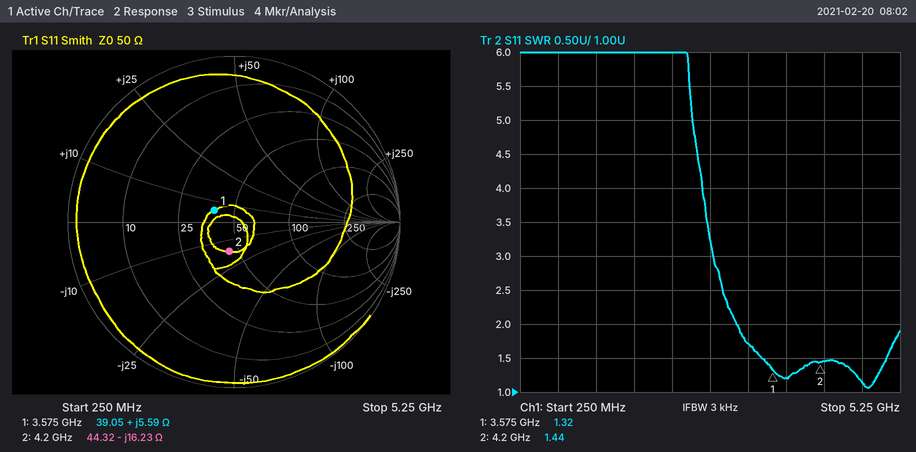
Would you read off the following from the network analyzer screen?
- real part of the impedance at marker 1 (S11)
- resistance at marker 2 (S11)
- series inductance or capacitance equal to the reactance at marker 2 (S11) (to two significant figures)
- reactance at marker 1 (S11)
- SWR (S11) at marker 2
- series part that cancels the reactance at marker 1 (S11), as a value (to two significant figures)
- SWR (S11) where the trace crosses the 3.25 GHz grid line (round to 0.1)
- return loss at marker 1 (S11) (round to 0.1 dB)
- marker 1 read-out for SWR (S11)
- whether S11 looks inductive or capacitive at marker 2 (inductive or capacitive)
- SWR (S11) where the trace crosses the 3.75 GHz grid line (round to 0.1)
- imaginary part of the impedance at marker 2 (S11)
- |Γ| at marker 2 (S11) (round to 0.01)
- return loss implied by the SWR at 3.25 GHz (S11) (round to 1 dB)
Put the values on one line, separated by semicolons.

39.05 Ω; 44.32 Ω; 2.3 pF; +5.59 Ω; 1.44; 8.0 pF; 1.7; 17.2 dB; 1.32; capacitive; 1.2; -16.23 Ω; 0.18; 12 dB
